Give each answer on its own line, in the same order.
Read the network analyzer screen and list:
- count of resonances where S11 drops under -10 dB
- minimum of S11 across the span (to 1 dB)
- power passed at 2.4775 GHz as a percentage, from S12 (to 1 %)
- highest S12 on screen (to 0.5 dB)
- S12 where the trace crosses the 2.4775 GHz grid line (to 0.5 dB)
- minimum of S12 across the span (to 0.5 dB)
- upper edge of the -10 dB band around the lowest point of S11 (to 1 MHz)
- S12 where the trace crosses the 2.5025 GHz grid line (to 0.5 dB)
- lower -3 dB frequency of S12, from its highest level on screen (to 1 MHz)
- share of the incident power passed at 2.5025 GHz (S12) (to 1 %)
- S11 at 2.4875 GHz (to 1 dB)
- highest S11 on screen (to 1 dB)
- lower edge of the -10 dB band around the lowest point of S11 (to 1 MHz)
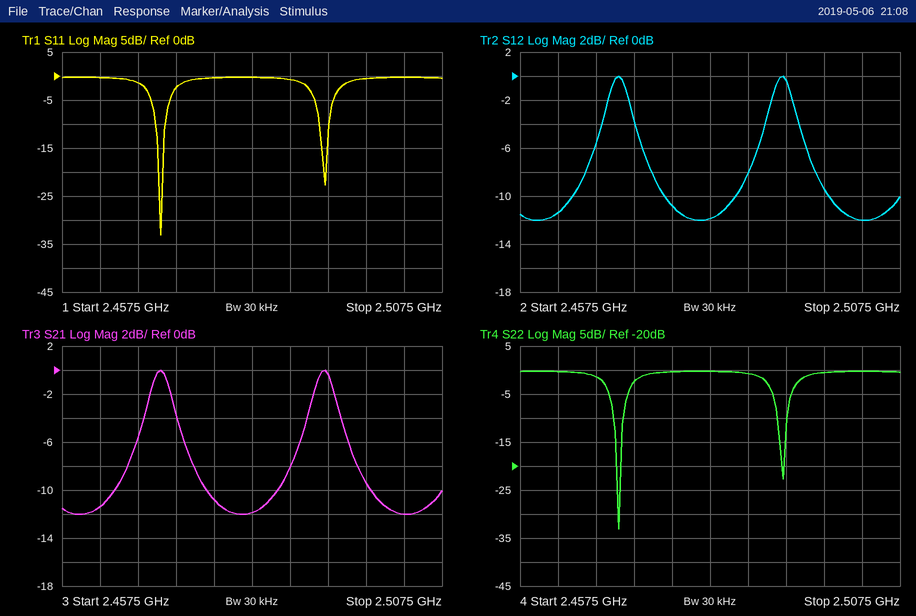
2
-33 dB
8 %
0.0 dB
-11.0 dB
-12.0 dB
2.471 GHz
-12.0 dB
2.469 GHz
6 %
-1 dB
0 dB
2.470 GHz
